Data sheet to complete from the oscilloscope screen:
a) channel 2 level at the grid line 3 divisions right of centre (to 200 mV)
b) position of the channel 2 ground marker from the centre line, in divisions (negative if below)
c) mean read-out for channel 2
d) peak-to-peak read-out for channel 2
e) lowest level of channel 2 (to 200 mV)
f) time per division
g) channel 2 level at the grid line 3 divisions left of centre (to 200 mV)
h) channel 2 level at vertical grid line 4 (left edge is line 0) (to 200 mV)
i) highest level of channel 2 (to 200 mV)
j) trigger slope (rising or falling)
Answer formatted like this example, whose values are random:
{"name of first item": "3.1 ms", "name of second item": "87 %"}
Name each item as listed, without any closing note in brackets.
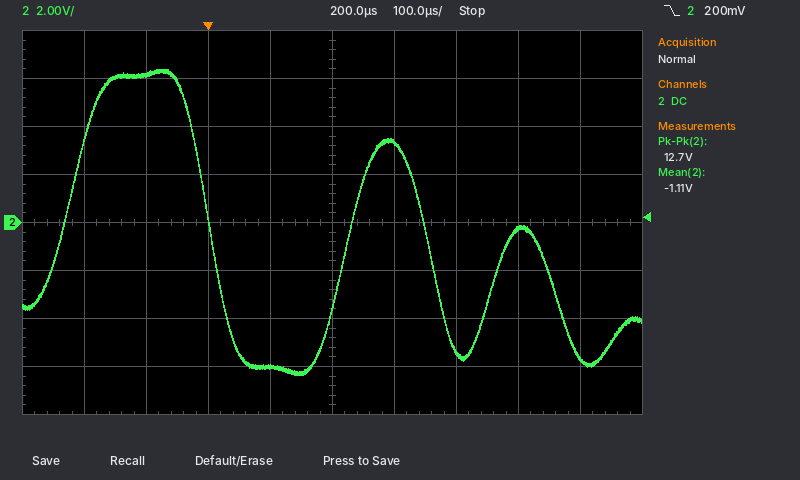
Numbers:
{"channel 2 level at the grid line 3 divisions right of centre": "-200 mV", "position of the channel 2 ground marker from the centre line, in divisions": "0.0 div", "mean read-out for channel 2": "-1.11 V", "peak-to-peak read-out for channel 2": "12.7 V", "lowest level of channel 2": "-6.4 V", "time per division": "100 µs", "channel 2 level at the grid line 3 divisions left of centre": "6.2 V", "channel 2 level at vertical grid line 4 (left edge is line 0)": "-6.0 V", "highest level of channel 2": "6.4 V", "trigger slope": "falling"}
